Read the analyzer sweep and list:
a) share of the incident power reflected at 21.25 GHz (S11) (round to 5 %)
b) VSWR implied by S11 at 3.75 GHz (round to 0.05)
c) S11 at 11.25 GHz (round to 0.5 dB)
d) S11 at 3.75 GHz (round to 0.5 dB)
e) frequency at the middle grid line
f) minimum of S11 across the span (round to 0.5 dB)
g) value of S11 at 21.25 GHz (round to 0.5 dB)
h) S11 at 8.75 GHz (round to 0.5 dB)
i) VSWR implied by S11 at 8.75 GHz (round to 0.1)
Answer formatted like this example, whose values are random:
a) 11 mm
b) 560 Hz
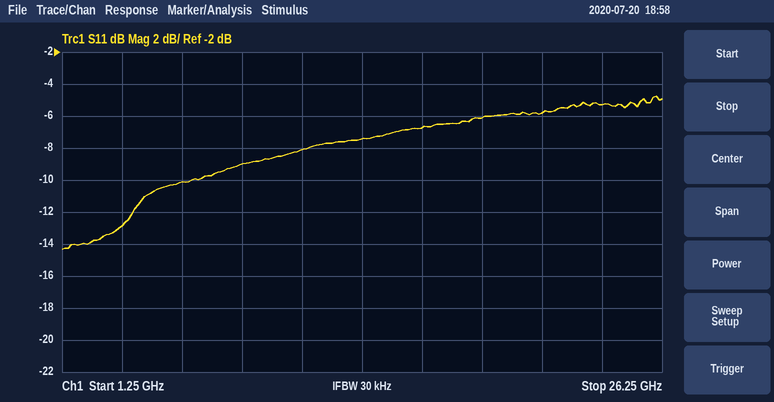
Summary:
a) 25 %
b) 1.60
c) -8.0 dB
d) -13.0 dB
e) 13.75 GHz
f) -14.5 dB
g) -6.0 dB
h) -9.0 dB
i) 2.1
